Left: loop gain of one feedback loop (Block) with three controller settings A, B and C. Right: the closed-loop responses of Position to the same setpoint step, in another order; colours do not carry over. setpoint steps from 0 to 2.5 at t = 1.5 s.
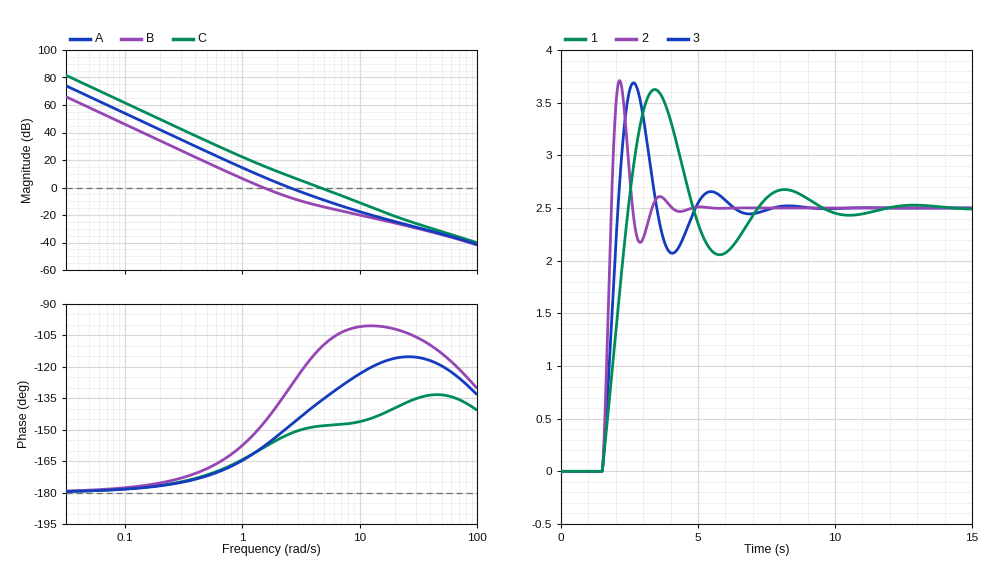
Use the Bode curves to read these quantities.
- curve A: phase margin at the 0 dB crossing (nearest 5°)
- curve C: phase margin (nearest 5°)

30°
30°
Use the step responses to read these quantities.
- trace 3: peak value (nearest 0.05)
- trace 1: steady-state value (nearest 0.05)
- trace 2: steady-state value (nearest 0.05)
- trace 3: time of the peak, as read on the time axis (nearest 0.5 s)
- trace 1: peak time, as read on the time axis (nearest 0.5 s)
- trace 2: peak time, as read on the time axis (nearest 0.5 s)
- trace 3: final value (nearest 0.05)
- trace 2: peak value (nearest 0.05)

3.70
2.50
2.50
2.5 s
3.5 s
2.0 s
2.50
3.70
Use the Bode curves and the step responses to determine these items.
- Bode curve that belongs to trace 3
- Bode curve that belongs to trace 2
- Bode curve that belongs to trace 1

A
C
B
